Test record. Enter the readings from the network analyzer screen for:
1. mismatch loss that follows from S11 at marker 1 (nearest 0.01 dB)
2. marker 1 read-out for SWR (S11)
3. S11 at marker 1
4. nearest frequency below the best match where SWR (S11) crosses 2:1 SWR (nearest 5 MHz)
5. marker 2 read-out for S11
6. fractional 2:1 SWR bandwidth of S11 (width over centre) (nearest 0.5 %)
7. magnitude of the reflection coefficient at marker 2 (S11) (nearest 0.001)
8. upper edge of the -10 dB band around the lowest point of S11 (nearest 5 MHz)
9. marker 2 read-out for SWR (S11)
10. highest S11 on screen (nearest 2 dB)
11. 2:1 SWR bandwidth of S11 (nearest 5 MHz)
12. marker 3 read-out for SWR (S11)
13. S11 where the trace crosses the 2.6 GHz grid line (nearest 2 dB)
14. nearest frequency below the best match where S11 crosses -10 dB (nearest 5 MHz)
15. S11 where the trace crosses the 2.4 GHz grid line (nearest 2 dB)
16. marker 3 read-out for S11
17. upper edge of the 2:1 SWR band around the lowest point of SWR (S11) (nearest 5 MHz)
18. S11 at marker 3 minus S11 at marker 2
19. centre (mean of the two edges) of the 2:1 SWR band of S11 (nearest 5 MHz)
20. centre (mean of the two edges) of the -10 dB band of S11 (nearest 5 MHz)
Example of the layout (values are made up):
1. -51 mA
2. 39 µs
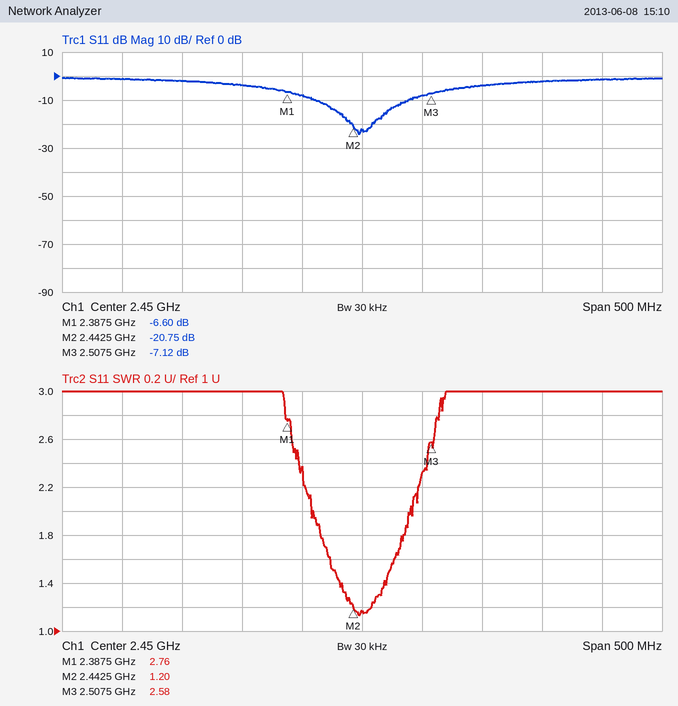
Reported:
1. 1.07 dB
2. 2.76
3. -6.60 dB
4. 2.410 GHz
5. -20.75 dB
6. 3.5 %
7. 0.092
8. 2.490 GHz
9. 1.20
10. 0 dB
11. 80 MHz
12. 2.58
13. -2 dB
14. 2.410 GHz
15. -8 dB
16. -7.12 dB
17. 2.490 GHz
18. 13.63 dB
19. 2.450 GHz
20. 2.450 GHz
